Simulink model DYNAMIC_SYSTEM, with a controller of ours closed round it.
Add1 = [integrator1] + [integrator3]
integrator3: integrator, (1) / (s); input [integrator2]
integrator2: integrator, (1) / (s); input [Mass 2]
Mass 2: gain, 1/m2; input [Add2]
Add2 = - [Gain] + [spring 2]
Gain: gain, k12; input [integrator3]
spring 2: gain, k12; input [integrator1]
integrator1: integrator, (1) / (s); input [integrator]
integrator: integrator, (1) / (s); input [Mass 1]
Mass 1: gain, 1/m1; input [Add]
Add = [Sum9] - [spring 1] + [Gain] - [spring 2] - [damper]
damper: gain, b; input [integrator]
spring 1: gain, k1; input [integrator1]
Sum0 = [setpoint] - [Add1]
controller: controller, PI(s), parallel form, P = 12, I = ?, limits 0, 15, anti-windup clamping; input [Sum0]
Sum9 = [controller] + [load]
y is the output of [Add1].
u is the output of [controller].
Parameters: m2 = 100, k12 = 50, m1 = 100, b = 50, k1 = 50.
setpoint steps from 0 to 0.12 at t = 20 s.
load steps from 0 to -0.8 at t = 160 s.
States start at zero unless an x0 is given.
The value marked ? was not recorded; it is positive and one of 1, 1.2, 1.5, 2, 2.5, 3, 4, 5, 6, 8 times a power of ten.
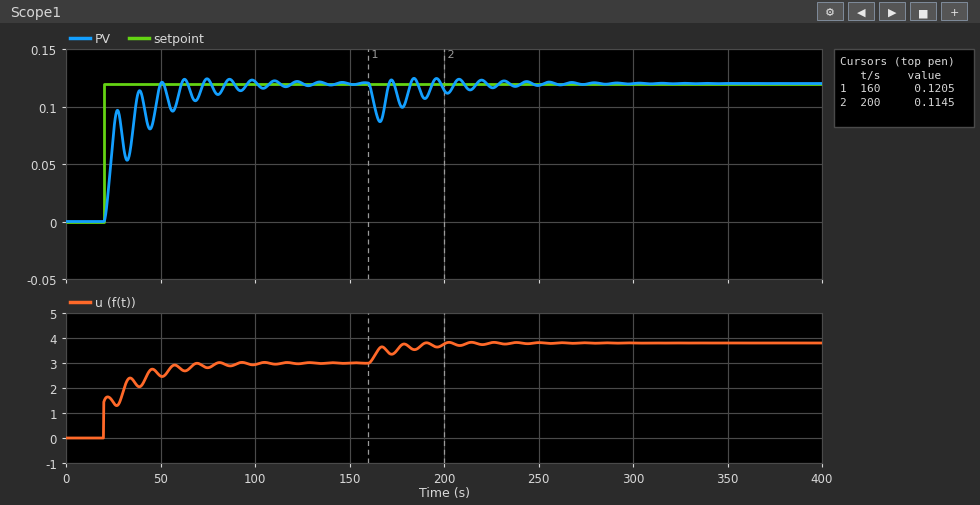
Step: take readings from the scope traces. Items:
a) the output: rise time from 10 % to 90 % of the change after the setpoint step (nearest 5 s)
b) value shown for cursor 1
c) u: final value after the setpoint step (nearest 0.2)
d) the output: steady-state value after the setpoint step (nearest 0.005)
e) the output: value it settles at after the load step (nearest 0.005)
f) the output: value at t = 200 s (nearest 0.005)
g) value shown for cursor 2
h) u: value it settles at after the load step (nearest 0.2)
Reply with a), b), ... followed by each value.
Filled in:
a) 15 s
b) 0.1205
c) 3.0
d) 0.120
e) 0.120
f) 0.115
g) 0.1145
h) 3.8
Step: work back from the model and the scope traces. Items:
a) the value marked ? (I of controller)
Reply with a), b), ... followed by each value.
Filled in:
a) 2
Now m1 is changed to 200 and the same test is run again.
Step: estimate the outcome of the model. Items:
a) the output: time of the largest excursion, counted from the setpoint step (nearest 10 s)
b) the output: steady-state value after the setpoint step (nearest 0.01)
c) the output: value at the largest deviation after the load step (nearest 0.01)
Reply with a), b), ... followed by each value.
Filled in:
a) 50 s
b) 0.12
c) 0.08
